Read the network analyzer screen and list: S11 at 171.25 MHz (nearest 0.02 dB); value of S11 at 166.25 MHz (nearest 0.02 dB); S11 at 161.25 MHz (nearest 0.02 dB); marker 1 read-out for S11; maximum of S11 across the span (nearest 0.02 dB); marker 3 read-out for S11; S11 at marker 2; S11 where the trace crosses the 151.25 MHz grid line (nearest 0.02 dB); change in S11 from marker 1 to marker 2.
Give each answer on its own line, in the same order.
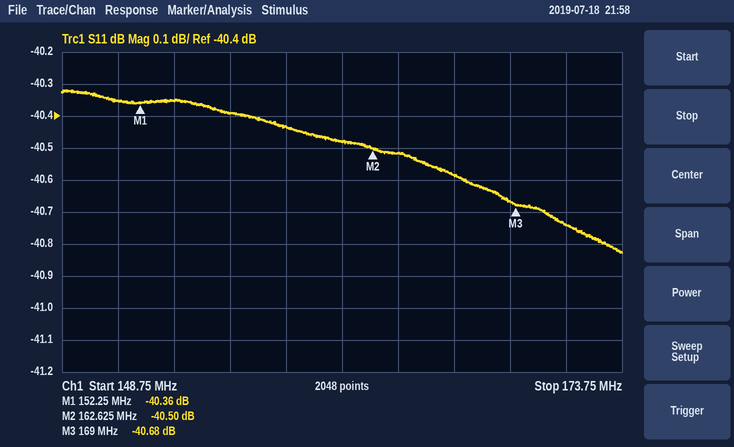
-40.74 dB
-40.58 dB
-40.48 dB
-40.36 dB
-40.32 dB
-40.68 dB
-40.50 dB
-40.36 dB
-0.14 dB
